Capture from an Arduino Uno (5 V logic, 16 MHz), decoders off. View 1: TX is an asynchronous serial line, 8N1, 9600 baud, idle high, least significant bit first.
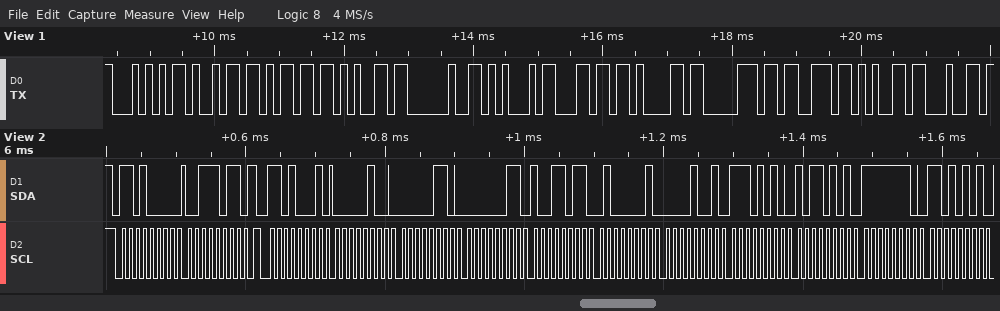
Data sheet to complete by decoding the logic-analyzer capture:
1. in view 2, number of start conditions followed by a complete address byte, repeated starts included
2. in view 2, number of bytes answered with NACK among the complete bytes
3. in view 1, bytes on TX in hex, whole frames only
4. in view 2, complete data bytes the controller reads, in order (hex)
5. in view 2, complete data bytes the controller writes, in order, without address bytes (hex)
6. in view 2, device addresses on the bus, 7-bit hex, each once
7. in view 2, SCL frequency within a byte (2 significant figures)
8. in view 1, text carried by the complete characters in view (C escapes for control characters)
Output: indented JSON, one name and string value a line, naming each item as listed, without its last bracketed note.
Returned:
{
  "in view 2, number of start conditions followed by a complete address byte, repeated starts included": "2",
  "in view 2, number of bytes answered with NACK among the complete bytes": "0",
  "in view 1, bytes on TX in hex, whole frames only": "54 69 6D 65 20 45 6C 61 70 73 65 64",
  "in view 2, complete data bytes the controller reads, in order": "04 06 03 9B 41 09 EA B5 FE D5",
  "in view 2, complete data bytes the controller writes, in order, without address bytes": "3B",
  "in view 2, device addresses on the bus, 7-bit hex, each once": "0x68",
  "in view 2, SCL frequency within a byte": "100 kHz",
  "in view 1, text carried by the complete characters in view": "\"Time Elapsed\""
}
